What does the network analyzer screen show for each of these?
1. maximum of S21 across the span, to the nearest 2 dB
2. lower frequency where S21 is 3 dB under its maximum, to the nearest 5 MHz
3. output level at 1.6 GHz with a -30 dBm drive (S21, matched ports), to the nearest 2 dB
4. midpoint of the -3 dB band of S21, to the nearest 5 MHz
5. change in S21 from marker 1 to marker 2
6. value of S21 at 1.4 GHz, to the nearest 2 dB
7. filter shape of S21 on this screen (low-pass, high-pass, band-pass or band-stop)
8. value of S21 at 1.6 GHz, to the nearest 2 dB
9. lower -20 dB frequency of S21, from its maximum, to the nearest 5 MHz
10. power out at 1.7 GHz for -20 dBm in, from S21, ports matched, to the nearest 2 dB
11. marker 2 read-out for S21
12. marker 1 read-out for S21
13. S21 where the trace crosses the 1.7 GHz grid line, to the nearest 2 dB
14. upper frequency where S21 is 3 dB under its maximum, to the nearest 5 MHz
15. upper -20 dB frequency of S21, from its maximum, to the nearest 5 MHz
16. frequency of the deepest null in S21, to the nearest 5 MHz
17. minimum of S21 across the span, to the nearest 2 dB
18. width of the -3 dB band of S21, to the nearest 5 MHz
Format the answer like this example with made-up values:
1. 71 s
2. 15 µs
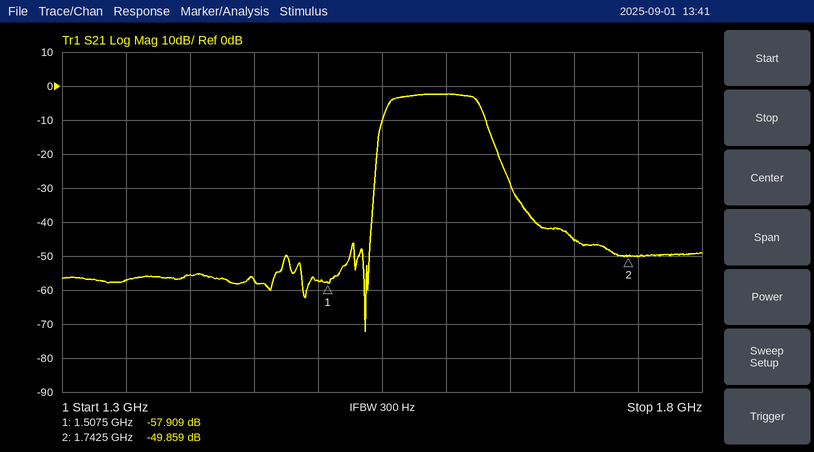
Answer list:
1. -2 dB
2. 1.555 GHz
3. -32 dBm
4. 1.590 GHz
5. 8.050 dB
6. -56 dB
7. band-pass
8. -2 dB
9. 1.545 GHz
10. -66 dBm
11. -49.859 dB
12. -57.909 dB
13. -46 dB
14. 1.625 GHz
15. 1.645 GHz
16. 1.535 GHz
17. -72 dB
18. 70 MHz
